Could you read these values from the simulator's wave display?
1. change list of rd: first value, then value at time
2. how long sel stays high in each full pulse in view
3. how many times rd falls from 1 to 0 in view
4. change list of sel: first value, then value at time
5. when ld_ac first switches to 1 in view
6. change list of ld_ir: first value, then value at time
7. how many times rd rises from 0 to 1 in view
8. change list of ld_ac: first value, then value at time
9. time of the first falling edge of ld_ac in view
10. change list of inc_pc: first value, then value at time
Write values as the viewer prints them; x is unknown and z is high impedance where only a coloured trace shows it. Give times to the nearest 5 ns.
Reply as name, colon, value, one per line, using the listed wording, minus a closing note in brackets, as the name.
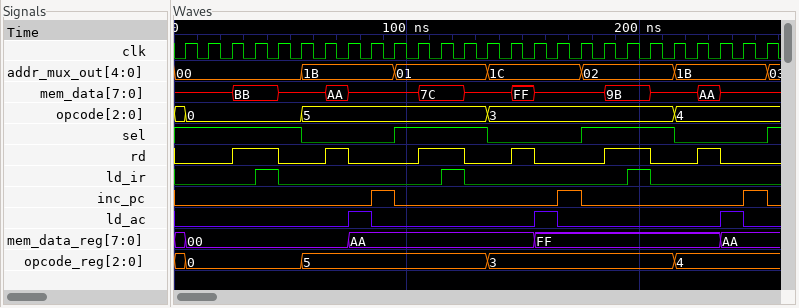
change list of rd: first value, then value at time: 0, 1 at 25 ns, 0 at 45 ns, 1 at 65 ns, 0 at 75 ns, 1 at 105 ns, 0 at 125 ns, 1 at 145 ns, 0 at 155 ns, 1 at 185 ns, 0 at 205 ns, 1 at 225 ns, 0 at 235 ns
how long sel stays high in each full pulse in view: 40 ns, 40 ns
how many times rd falls from 1 to 0 in view: 6
change list of sel: first value, then value at time: 1, 0 at 55 ns, 1 at 95 ns, 0 at 135 ns, 1 at 175 ns, 0 at 215 ns, 1 at 255 ns
when ld_ac first switches to 1 in view: 75 ns
change list of ld_ir: first value, then value at time: 0, 1 at 35 ns, 0 at 45 ns, 1 at 115 ns, 0 at 125 ns, 1 at 195 ns, 0 at 205 ns
how many times rd rises from 0 to 1 in view: 6
change list of ld_ac: first value, then value at time: 0, 1 at 75 ns, 0 at 85 ns, 1 at 155 ns, 0 at 165 ns, 1 at 235 ns, 0 at 245 ns
time of the first falling edge of ld_ac in view: 85 ns
change list of inc_pc: first value, then value at time: 0, 1 at 85 ns, 0 at 95 ns, 1 at 165 ns, 0 at 175 ns, 1 at 245 ns, 0 at 255 ns
